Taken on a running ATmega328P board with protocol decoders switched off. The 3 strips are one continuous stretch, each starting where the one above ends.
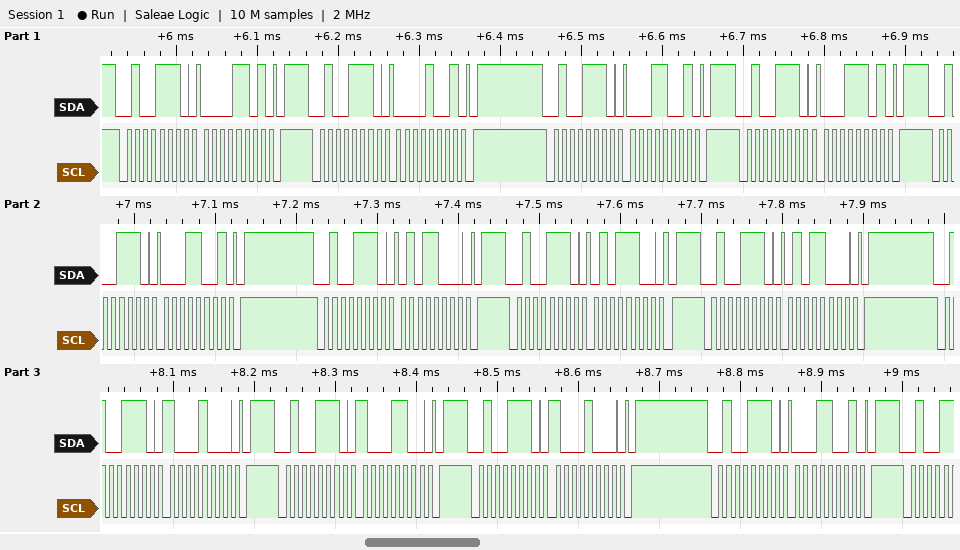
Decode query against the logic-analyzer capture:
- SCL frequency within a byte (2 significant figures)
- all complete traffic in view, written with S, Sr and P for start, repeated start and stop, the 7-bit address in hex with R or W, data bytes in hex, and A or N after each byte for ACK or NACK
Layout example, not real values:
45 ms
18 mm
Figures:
100 kHz
S 27W A 0D A P S 27W A 09 A P S 27W A 19 A P S 27W A 1D A P S 27W A 19 A P S 27W A 58 A P S 27W A 5C A P S 27W A 58 A P S 27W A 88 A P S 27W A 8C A P S 27W A 88 A P S 27W A 19 A P
